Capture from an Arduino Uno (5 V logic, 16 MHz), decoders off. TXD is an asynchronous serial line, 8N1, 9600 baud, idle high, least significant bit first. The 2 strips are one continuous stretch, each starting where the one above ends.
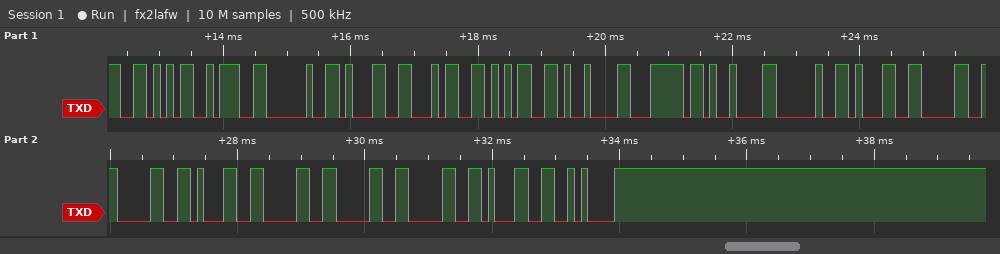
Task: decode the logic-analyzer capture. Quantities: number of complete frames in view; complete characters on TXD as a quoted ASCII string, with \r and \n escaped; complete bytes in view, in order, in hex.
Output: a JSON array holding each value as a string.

["19", "\"V: 145\\t|\\t 10010001\\n\"", "0x56 0x3A 0x20 0x31 0x34 0x35 0x09 0x7C 0x09 0x20 0x31 0x30 0x30 0x31 0x30 0x30 0x30 0x31 0x0A"]
